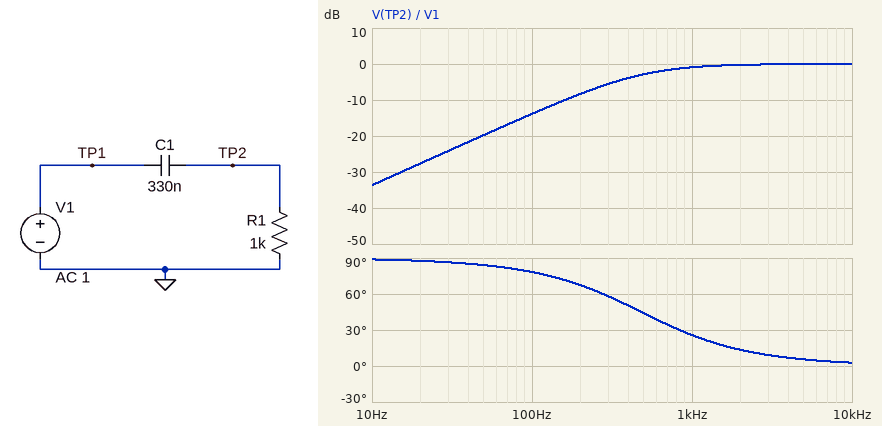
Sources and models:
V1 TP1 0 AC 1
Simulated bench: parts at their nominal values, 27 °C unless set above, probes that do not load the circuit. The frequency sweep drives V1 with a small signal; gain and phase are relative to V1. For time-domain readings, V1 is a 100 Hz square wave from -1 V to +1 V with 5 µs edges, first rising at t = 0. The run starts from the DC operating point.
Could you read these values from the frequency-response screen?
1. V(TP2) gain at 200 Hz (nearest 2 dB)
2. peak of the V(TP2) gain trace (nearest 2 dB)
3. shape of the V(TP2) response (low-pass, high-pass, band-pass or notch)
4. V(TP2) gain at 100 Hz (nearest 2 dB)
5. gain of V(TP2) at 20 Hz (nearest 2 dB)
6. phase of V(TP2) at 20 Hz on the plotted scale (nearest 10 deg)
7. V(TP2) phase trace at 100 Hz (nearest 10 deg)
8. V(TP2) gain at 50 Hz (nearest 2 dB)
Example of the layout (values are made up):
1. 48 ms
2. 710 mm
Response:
1. -8 dB
2. 0 dB
3. high-pass
4. -14 dB
5. -28 dB
6. 90 deg
7. 80 deg
8. -20 dB
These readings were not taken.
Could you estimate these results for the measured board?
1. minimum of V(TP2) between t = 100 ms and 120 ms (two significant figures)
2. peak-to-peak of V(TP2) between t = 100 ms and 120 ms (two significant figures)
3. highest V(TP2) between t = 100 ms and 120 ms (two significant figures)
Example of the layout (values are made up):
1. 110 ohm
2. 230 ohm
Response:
1. -2.0 V
2. 4.0 V
3. 2.0 V
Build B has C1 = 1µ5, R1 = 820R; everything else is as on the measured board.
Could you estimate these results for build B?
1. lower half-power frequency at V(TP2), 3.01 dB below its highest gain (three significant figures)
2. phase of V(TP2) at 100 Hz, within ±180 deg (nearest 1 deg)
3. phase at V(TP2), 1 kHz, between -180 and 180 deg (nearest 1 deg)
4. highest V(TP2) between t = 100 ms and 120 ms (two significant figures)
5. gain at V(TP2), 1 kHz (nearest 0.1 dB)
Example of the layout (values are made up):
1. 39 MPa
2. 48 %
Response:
1. 129 Hz
2. 52 deg
3. 7 deg
4. 2.0 V
5. -0.1 dB
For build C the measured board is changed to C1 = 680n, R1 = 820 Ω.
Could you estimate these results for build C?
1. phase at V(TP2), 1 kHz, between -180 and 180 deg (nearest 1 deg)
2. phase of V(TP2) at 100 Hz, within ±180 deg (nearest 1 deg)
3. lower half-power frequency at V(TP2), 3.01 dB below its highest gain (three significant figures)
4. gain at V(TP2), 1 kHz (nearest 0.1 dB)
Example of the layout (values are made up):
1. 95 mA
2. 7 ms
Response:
1. 16 deg
2. 71 deg
3. 285 Hz
4. -0.3 dB
